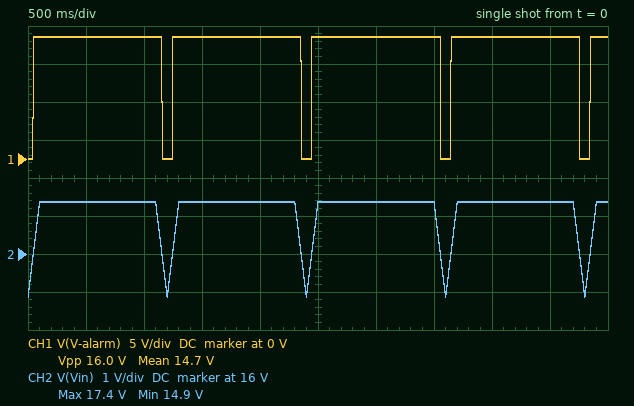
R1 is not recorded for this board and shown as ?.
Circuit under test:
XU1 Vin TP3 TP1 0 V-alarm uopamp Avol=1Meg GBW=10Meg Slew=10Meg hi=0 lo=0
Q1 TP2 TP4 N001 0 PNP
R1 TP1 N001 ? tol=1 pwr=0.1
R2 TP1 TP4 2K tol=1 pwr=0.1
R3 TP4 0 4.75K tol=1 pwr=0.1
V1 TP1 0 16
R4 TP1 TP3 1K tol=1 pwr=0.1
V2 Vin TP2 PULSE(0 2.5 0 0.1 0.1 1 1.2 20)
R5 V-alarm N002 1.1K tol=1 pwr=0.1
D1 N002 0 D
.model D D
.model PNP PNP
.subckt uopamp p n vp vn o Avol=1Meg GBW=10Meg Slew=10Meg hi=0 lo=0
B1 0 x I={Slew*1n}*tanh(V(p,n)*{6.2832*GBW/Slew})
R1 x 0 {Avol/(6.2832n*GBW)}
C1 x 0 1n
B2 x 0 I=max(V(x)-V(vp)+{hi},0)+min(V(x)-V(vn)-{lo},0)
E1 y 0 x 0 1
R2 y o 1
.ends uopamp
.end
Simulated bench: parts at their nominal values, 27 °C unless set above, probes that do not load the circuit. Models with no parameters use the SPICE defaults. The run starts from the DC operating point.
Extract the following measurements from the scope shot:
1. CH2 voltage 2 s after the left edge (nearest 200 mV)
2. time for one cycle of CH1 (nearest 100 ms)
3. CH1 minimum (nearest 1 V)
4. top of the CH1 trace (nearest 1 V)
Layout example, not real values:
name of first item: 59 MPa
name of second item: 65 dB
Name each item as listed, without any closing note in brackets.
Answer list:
CH2 voltage 2 s after the left edge: 17.4 V
time for one cycle of CH1: 1.2 s
CH1 minimum: 0 V
top of the CH1 trace: 16 V
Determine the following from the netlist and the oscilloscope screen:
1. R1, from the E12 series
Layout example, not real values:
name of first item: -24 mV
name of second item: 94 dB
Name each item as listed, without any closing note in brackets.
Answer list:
R1, from the E12 series: 560 Ω
